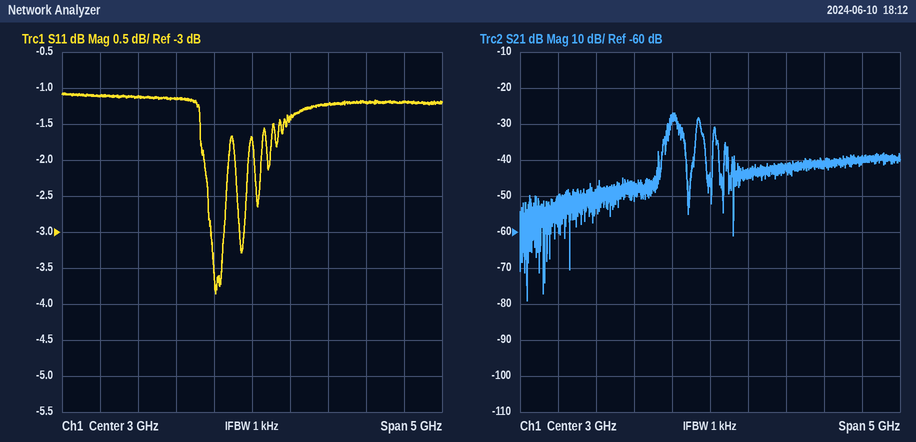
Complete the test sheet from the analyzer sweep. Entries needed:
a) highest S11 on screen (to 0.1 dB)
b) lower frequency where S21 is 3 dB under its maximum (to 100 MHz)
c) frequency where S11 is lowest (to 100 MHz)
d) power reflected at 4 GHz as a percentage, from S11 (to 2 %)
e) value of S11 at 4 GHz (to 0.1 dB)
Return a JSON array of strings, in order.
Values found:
["-1.1 dB", "2.5 GHz", "2.5 GHz", "76 %", "-1.2 dB"]
